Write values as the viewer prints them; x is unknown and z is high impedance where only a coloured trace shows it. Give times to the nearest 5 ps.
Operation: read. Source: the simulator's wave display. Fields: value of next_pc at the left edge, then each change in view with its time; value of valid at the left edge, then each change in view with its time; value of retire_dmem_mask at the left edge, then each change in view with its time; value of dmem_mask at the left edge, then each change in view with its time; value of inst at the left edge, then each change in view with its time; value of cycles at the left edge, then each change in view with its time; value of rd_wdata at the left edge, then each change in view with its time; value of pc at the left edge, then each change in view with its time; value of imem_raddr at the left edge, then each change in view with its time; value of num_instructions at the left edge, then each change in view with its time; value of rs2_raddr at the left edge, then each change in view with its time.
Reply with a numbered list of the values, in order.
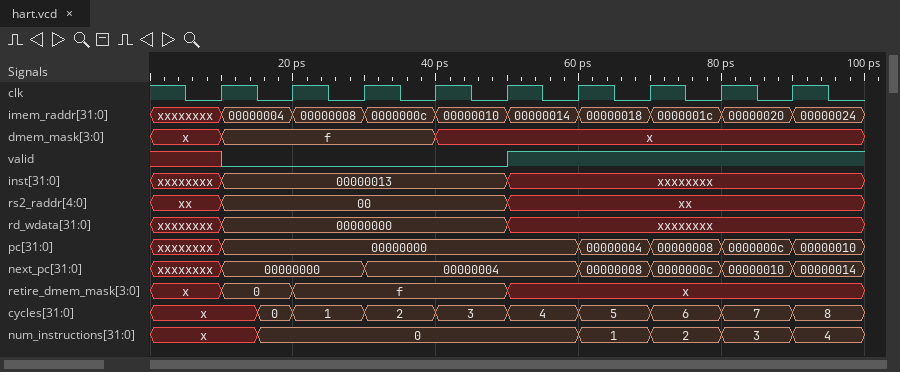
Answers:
1. xxxxxxxx, 00000000 at 10 ps, 00000004 at 30 ps, 00000008 at 60 ps, 0000000c at 70 ps, 00000010 at 80 ps, 00000014 at 90 ps
2. x, 0 at 10 ps, 1 at 50 ps
3. x, 0 at 10 ps, f at 20 ps, x at 50 ps
4. x, f at 10 ps, x at 40 ps
5. xxxxxxxx, 00000013 at 10 ps, xxxxxxxx at 50 ps
6. x, 0 at 15 ps, 1 at 20 ps, 2 at 30 ps, 3 at 40 ps, 4 at 50 ps, 5 at 60 ps, 6 at 70 ps, 7 at 80 ps, 8 at 90 ps
7. xxxxxxxx, 00000000 at 10 ps, xxxxxxxx at 50 ps
8. xxxxxxxx, 00000000 at 10 ps, 00000004 at 60 ps, 00000008 at 70 ps, 0000000c at 80 ps, 00000010 at 90 ps
9. xxxxxxxx, 00000004 at 10 ps, 00000008 at 20 ps, 0000000c at 30 ps, 00000010 at 40 ps, 00000014 at 50 ps, 00000018 at 60 ps, 0000001c at 70 ps, 00000020 at 80 ps, 00000024 at 90 ps
10. x, 0 at 15 ps, 1 at 60 ps, 2 at 70 ps, 3 at 80 ps, 4 at 90 ps
11. xx, 00 at 10 ps, xx at 50 ps
